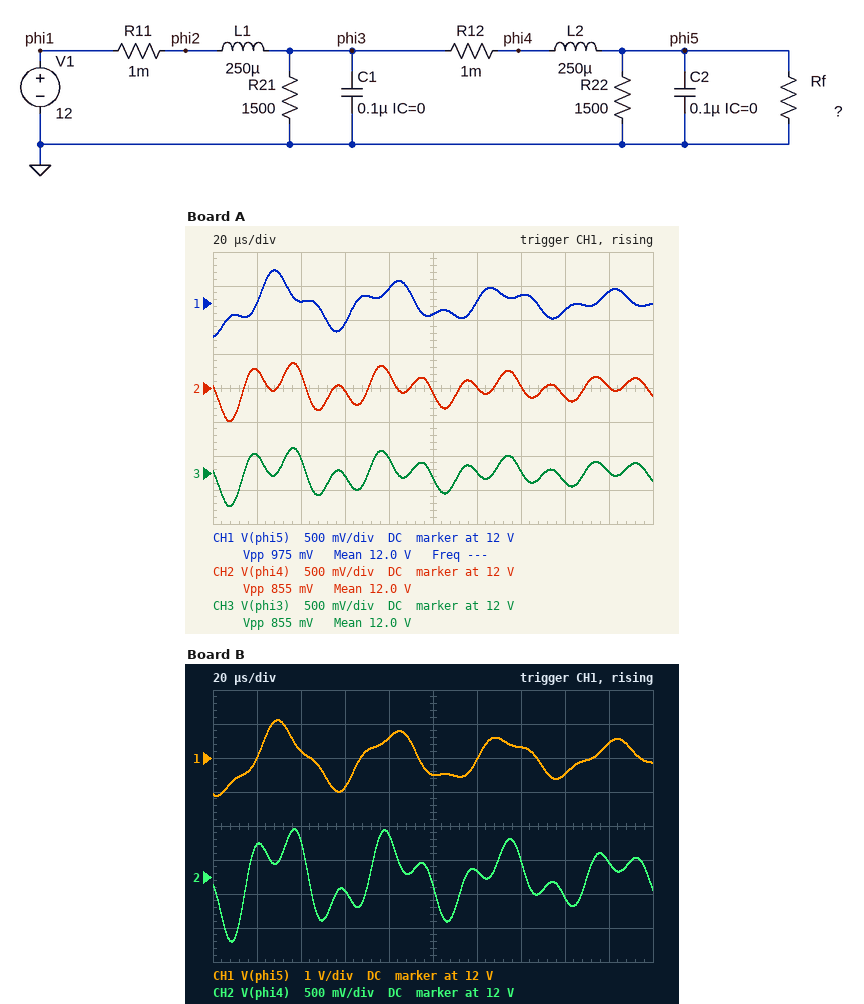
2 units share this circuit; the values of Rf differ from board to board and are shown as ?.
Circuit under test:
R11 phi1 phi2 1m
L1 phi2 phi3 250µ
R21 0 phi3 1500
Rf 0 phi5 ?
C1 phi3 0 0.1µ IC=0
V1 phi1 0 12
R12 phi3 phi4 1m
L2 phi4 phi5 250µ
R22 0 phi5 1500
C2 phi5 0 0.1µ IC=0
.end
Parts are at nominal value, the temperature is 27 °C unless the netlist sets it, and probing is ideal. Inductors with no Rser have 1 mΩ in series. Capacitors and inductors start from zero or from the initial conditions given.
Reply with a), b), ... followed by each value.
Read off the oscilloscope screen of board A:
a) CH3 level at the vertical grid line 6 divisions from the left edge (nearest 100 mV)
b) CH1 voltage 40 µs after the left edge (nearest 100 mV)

a) 12.0 V
b) 12.0 V
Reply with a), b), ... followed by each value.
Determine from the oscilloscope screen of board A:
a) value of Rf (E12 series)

a) 1.2 kΩ
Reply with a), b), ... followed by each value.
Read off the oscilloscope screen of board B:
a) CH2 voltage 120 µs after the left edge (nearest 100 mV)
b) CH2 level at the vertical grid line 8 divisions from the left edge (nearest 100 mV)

a) 12.1 V
b) 11.7 V
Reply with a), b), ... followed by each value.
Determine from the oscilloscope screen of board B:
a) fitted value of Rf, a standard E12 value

a) 2.7 kΩ
